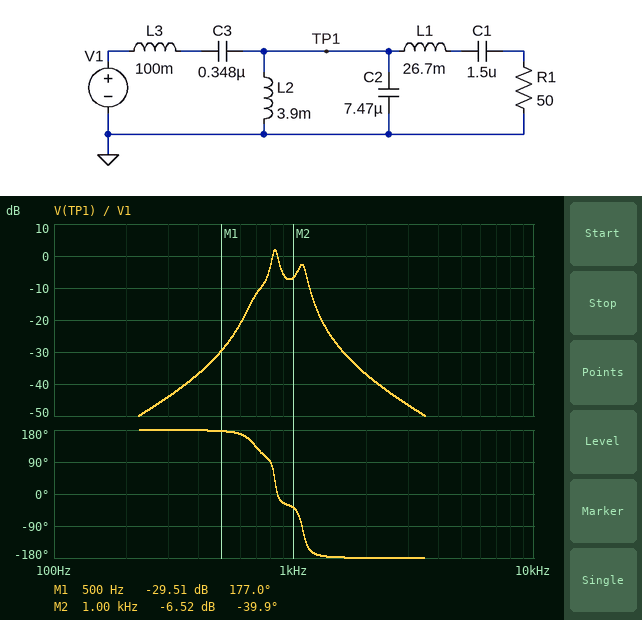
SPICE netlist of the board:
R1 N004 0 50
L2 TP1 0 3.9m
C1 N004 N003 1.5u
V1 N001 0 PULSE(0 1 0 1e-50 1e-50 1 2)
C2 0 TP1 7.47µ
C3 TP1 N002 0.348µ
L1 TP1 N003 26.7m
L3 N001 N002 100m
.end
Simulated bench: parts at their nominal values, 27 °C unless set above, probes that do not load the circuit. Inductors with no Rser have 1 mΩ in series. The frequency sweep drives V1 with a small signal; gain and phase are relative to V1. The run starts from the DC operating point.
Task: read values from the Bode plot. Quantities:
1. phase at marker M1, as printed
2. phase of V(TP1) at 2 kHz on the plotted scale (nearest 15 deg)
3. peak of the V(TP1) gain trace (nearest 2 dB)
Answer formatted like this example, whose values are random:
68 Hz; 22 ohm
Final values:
177.0 deg; -180 deg; 2 dB
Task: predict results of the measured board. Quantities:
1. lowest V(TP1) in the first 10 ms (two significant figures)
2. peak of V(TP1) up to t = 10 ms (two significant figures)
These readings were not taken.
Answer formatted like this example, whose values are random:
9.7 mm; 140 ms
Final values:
-95 mV; 100 mV
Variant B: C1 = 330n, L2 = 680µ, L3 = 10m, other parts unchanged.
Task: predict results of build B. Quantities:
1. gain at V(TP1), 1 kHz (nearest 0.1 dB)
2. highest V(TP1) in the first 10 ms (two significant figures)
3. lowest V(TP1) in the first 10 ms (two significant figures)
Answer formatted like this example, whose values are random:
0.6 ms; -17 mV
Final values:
-37.1 dB; 160 mV; -180 mV
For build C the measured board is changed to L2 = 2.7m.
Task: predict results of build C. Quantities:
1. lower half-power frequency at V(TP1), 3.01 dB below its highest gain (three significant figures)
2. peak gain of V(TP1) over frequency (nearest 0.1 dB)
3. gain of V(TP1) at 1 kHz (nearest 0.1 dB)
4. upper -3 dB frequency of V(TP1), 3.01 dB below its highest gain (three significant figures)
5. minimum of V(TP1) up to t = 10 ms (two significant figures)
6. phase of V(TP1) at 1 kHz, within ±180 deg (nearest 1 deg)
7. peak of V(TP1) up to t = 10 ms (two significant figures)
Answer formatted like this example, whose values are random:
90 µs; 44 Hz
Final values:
828 Hz; 6.8 dB; -13.8 dB; 845 Hz; -65 mV; -16 deg; 74 mV
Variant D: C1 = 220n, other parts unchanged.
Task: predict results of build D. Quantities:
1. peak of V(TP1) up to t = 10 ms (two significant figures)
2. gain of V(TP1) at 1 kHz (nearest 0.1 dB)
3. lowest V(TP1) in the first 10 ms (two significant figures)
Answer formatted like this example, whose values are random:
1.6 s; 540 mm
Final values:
190 mV; 9.0 dB; -180 mV
